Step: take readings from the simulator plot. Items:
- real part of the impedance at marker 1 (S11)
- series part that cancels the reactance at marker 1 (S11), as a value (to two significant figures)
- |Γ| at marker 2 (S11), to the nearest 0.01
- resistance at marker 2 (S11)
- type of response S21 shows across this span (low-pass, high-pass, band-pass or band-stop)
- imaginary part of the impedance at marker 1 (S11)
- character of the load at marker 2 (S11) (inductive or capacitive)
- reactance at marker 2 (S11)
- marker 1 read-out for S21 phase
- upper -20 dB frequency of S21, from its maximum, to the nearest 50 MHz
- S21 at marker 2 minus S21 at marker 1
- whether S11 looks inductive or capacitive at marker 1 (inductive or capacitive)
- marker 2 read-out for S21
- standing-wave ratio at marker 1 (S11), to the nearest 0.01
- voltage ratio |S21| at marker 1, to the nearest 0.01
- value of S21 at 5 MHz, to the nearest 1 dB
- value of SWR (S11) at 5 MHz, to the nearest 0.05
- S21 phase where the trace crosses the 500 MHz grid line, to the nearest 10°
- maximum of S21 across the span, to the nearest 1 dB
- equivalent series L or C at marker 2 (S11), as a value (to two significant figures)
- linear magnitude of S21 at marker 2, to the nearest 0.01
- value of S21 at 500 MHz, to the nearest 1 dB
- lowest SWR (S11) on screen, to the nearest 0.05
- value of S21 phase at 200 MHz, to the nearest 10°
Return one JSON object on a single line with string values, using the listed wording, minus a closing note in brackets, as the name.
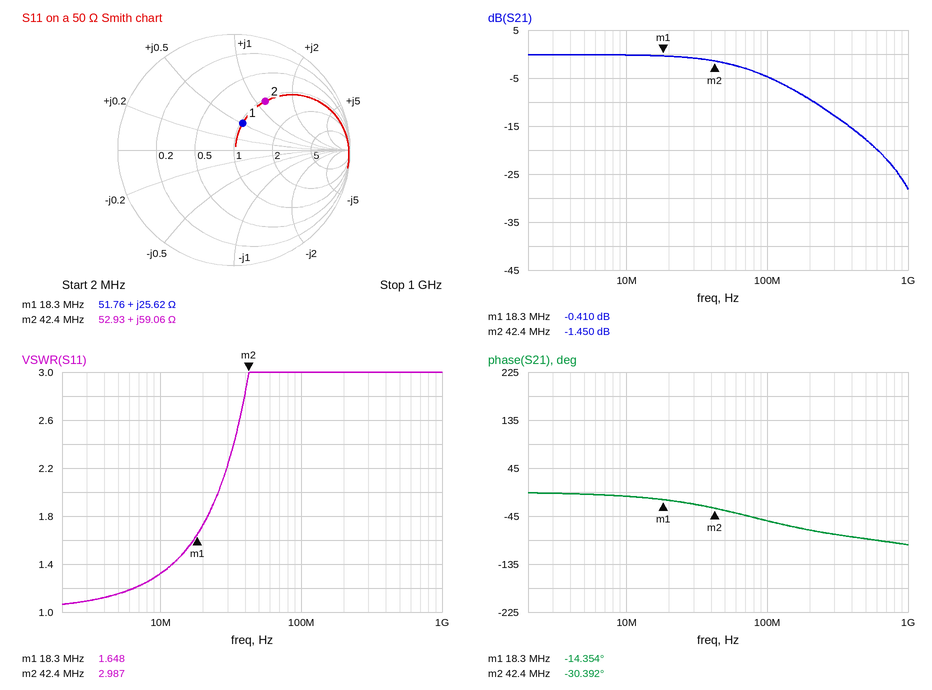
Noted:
{"real part of the impedance at marker 1": "51.76 Ω", "series part that cancels the reactance at marker 1 (S11), as a value": "340 pF", "|Γ| at marker 2 (S11), to the nearest 0.01": "0.50", "resistance at marker 2": "52.93 Ω", "type of response S21 shows across this span": "low-pass", "imaginary part of the impedance at marker 1": "+25.62 Ω", "character of the load at marker 2 (S11)": "inductive", "reactance at marker 2": "+59.06 Ω", "marker 1 read-out for S21 phase": "-14.354°", "upper -20 dB frequency of S21, from its maximum, to the nearest 50 MHz": "600 MHz", "S21 at marker 2 minus S21 at marker 1": "-1.040 dB", "whether S11 looks inductive or capacitive at marker 1": "inductive", "marker 2 read-out for S21": "-1.450 dB", "standing-wave ratio at marker 1 (S11), to the nearest 0.01": "1.65", "voltage ratio |S21| at marker 1, to the nearest 0.01": "0.95", "value of S21 at 5 MHz, to the nearest 1 dB": "0 dB", "value of SWR (S11) at 5 MHz, to the nearest 0.05": "1.15", "S21 phase where the trace crosses the 500 MHz grid line, to the nearest 10°": "-90°", "maximum of S21 across the span, to the nearest 1 dB": "0 dB", "equivalent series L or C at marker 2 (S11), as a value": "220 nH", "linear magnitude of S21 at marker 2, to the nearest 0.01": "0.85", "value of S21 at 500 MHz, to the nearest 1 dB": "-18 dB", "lowest SWR (S11) on screen, to the nearest 0.05": "1.05", "value of S21 phase at 200 MHz, to the nearest 10°": "-70°"}
